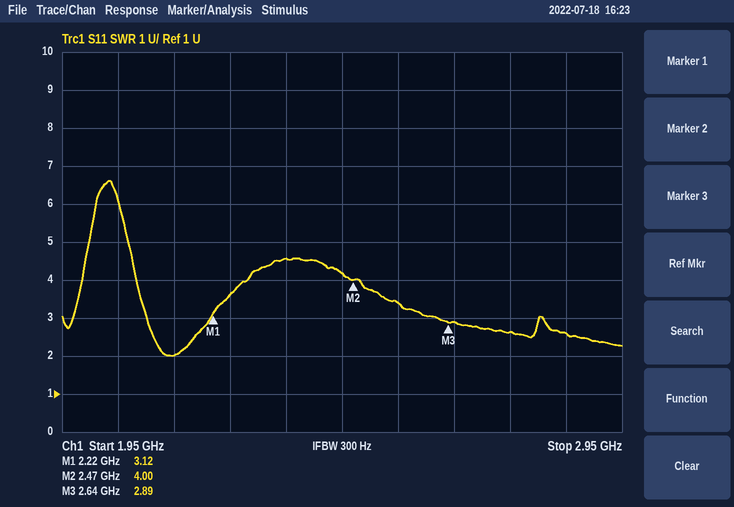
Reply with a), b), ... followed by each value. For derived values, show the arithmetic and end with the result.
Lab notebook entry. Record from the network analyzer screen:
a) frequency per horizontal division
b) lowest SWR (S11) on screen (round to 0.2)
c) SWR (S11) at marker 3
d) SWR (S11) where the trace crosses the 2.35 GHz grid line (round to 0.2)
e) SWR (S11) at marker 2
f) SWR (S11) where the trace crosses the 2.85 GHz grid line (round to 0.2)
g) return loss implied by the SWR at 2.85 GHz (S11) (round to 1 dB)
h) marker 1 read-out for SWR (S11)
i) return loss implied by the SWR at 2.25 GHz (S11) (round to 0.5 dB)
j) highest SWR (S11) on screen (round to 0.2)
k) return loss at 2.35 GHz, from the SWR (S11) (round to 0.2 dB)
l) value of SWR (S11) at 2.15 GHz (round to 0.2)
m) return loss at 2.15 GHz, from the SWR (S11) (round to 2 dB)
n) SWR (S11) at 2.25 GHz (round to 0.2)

a) 100 MHz
b) 2.0
c) 2.89
d) 4.6
e) 4.00
f) 2.6
g) −20 log10((2.6 − 1)/(2.6 + 1)) ≈ 7 dB
h) 3.12
i) −20 log10((3.6 − 1)/(3.6 + 1)) ≈ 5.0 dB
j) 6.6
k) −20 log10((4.6 − 1)/(4.6 + 1)) ≈ 3.8 dB
l) 2.0
m) −20 log10((2 − 1)/(2 + 1)) ≈ 10 dB
n) 3.6
